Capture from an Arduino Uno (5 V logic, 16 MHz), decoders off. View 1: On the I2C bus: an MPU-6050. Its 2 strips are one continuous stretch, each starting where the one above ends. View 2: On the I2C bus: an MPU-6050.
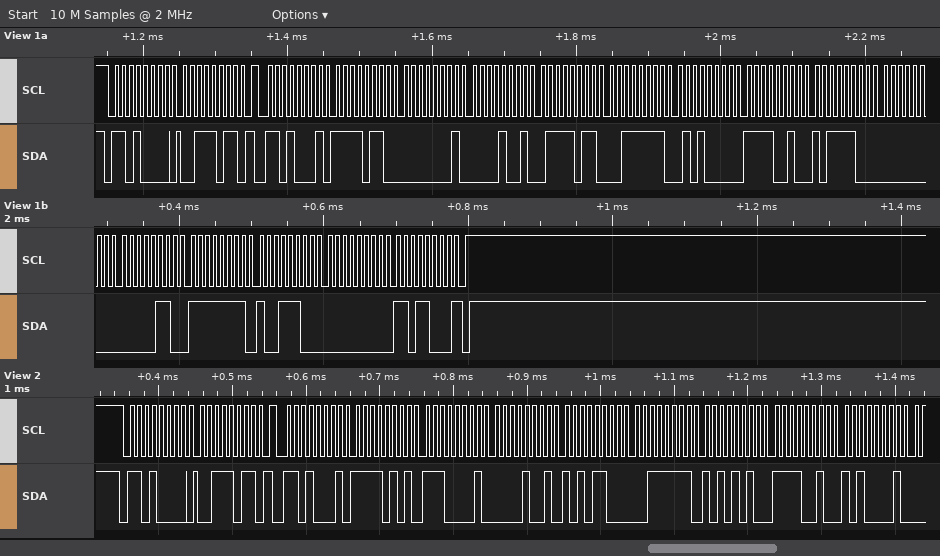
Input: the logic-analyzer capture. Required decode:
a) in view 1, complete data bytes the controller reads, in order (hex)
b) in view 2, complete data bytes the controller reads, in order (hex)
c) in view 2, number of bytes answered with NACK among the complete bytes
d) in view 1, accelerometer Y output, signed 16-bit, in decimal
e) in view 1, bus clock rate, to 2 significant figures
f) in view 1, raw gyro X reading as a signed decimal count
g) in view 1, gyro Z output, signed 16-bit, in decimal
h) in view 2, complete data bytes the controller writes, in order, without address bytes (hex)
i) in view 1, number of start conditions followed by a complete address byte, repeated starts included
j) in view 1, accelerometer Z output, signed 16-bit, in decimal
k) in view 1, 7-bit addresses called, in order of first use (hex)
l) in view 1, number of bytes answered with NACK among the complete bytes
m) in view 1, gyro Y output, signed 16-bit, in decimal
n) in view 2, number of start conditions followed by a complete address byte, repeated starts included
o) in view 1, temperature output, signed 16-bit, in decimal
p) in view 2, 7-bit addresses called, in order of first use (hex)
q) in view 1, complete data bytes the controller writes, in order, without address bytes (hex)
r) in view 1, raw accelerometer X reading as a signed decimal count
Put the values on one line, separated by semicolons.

F6 01 09 7B 3F 50 F2 BC 00 06 FF 9C 00 D8; F5 E1 09 AC 3F AA F2 A1; 0; 2427; 100 kHz; 6; 216; 3B; 2; 16208; 0x68; 1; -100; 2; -3396; 0x68; 3B; -2559
